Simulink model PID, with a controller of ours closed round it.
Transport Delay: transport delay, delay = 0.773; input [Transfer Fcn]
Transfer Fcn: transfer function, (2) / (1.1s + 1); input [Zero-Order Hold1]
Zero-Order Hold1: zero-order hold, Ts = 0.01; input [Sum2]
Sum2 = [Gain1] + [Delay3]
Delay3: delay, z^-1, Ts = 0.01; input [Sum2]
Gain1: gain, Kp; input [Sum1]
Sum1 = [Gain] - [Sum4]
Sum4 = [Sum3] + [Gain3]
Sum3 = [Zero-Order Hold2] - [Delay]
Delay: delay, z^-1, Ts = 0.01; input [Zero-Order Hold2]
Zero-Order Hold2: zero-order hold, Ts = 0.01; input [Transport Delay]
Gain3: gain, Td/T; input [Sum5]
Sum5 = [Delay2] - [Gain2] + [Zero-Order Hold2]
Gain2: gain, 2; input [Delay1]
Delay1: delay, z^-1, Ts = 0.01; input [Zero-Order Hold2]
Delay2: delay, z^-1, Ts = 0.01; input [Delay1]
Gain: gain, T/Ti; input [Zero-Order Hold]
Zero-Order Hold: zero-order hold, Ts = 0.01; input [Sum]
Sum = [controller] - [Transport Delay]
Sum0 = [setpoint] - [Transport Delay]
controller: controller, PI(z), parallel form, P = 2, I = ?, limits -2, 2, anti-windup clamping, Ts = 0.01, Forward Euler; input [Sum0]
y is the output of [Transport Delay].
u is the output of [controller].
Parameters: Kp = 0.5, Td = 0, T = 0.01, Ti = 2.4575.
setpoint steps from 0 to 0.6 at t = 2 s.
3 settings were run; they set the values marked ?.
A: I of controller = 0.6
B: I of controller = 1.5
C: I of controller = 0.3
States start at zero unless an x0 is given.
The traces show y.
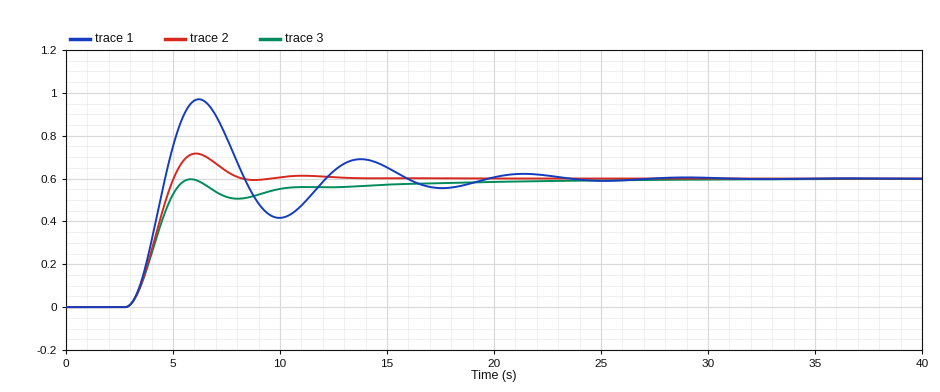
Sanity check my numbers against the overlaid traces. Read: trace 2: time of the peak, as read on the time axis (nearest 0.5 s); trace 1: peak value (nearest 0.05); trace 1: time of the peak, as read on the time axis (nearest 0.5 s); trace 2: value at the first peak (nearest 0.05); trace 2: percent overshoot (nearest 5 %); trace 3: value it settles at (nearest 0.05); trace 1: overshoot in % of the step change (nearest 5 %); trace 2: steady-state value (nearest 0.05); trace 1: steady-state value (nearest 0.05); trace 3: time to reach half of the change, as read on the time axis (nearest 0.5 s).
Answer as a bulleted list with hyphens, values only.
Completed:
- 6.0 s
- 0.95
- 6.0 s
- 0.70
- 20 %
- 0.60
- 60 %
- 0.60
- 0.60
- 4.0 s
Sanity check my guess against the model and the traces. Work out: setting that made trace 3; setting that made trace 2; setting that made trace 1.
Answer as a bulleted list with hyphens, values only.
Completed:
- C
- A
- B
